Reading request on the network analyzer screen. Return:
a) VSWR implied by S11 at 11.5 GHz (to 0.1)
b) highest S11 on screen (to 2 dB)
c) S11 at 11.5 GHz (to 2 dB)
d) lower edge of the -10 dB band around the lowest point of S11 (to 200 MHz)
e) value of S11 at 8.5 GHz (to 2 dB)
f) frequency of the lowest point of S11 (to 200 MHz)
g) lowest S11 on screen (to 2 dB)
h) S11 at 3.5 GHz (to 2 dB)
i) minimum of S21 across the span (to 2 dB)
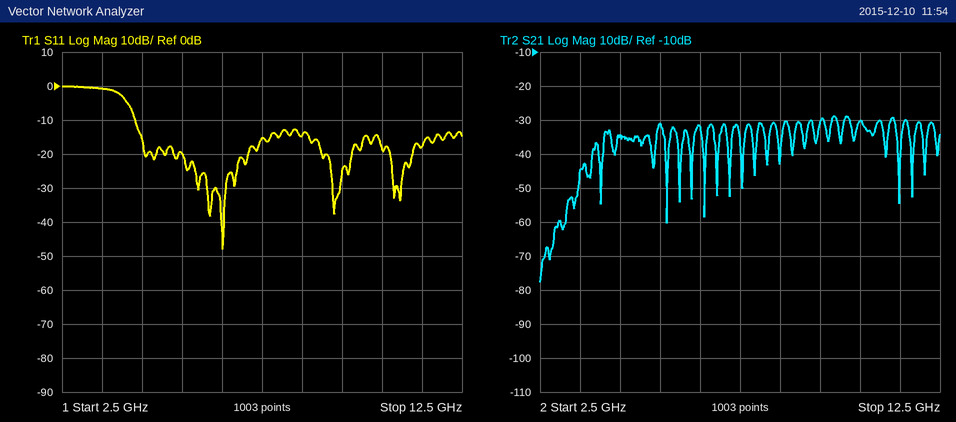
1.3
0 dB
-18 dB
4.4 GHz
-14 dB
6.6 GHz
-48 dB
0 dB
-78 dB
